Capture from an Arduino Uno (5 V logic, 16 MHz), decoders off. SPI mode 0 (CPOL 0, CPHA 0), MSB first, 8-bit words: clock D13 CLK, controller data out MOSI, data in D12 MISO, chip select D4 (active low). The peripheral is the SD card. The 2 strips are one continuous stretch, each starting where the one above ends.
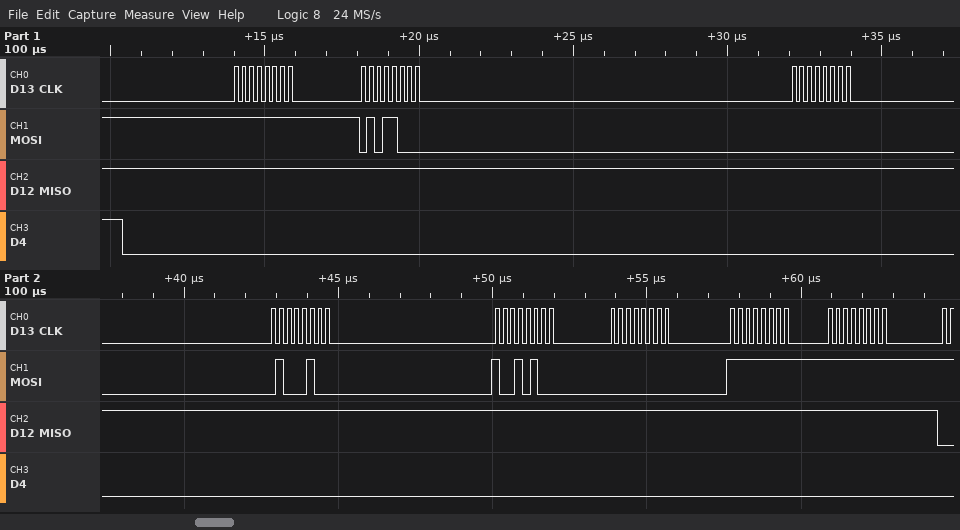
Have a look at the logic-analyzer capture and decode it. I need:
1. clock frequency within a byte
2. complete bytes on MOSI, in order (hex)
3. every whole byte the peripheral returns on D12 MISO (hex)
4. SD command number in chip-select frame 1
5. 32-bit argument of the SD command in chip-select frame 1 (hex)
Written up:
4 MHz
FF 58 00 44 94 00 FF FF
FF FF FF FF FF FF FF FF
CMD24
0x00449400
